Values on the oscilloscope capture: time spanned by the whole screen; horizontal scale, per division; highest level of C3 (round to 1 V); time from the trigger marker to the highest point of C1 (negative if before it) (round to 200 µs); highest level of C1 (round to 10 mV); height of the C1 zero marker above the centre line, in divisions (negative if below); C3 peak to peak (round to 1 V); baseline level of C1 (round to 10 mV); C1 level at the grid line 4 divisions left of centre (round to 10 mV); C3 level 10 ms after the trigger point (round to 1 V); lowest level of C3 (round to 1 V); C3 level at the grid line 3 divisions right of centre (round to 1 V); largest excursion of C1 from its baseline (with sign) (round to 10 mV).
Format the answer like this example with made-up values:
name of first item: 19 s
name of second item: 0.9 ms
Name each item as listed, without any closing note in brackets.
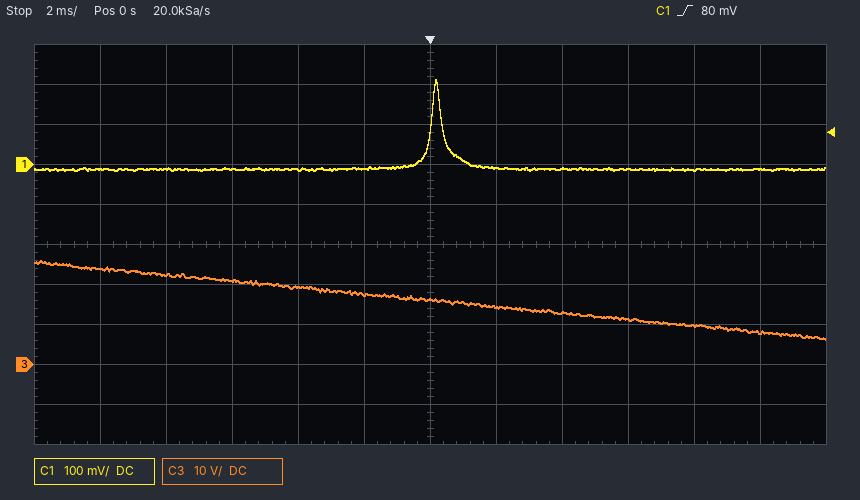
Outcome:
time spanned by the whole screen: 24 ms
horizontal scale, per division: 2 ms
highest level of C3: 26 V
time from the trigger marker to the highest point of C1 (negative if before it): +200 µs
highest level of C1: 210 mV
height of the C1 zero marker above the centre line, in divisions: +2.0 div
C3 peak to peak: 20 V
baseline level of C1: -10 mV
C1 level at the grid line 4 divisions left of centre: -10 mV
C3 level 10 ms after the trigger point: 8 V
lowest level of C3: 6 V
C3 level at the grid line 3 divisions right of centre: 11 V
largest excursion of C1 from its baseline (with sign): +220 mV
